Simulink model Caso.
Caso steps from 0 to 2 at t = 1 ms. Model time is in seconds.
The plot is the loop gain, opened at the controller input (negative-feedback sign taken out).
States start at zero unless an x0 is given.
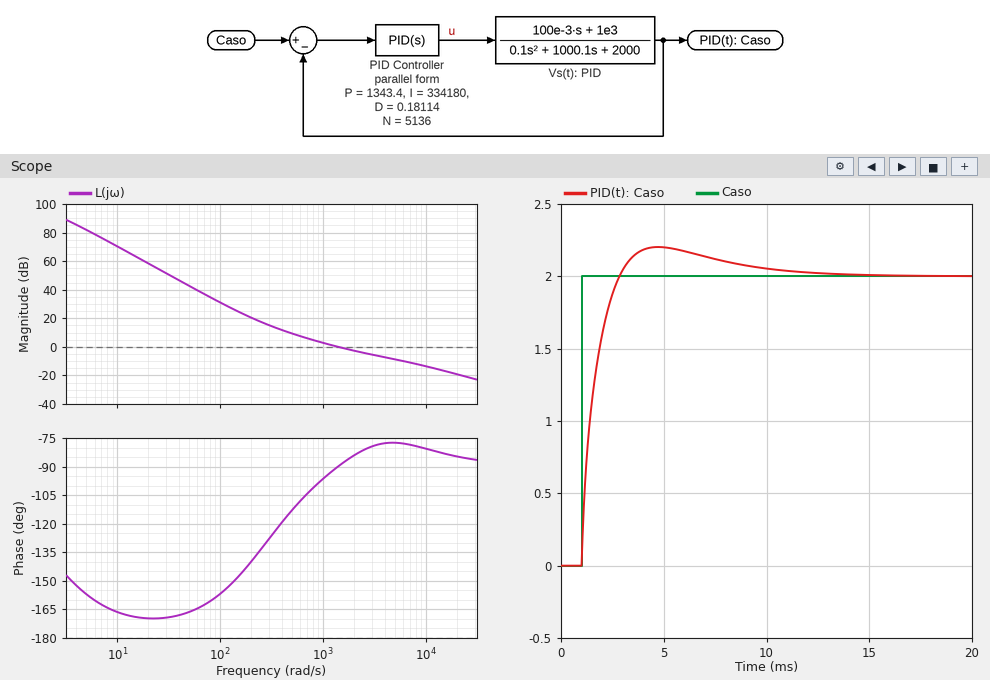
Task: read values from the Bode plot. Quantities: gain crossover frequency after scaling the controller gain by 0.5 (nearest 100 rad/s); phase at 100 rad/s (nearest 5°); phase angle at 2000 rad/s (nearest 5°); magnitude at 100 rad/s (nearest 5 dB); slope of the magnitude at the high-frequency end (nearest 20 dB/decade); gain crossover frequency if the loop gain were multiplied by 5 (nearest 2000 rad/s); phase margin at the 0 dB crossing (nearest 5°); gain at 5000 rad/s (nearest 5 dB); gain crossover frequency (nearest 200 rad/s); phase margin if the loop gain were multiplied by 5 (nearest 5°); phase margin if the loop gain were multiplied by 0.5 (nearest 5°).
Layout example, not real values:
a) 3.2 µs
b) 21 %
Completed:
a) 700 rad/s
b) -155°
c) -85°
d) 30 dB
e) -20 dB/decade
f) 10000 rad/s
g) 90°
h) -10 dB
i) 1400 rad/s
j) 100°
k) 75°
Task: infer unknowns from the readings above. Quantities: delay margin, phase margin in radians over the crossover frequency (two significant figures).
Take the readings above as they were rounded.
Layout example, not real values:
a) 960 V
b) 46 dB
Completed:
a) 0.0011 s
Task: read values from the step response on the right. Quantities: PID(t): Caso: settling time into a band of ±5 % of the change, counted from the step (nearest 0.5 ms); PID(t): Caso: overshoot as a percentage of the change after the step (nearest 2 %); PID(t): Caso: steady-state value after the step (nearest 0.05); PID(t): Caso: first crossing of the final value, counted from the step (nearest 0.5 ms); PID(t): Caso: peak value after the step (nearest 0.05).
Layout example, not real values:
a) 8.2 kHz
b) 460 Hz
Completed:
a) 7.0 ms
b) 10 %
c) 2.00
d) 2.0 ms
e) 2.20
